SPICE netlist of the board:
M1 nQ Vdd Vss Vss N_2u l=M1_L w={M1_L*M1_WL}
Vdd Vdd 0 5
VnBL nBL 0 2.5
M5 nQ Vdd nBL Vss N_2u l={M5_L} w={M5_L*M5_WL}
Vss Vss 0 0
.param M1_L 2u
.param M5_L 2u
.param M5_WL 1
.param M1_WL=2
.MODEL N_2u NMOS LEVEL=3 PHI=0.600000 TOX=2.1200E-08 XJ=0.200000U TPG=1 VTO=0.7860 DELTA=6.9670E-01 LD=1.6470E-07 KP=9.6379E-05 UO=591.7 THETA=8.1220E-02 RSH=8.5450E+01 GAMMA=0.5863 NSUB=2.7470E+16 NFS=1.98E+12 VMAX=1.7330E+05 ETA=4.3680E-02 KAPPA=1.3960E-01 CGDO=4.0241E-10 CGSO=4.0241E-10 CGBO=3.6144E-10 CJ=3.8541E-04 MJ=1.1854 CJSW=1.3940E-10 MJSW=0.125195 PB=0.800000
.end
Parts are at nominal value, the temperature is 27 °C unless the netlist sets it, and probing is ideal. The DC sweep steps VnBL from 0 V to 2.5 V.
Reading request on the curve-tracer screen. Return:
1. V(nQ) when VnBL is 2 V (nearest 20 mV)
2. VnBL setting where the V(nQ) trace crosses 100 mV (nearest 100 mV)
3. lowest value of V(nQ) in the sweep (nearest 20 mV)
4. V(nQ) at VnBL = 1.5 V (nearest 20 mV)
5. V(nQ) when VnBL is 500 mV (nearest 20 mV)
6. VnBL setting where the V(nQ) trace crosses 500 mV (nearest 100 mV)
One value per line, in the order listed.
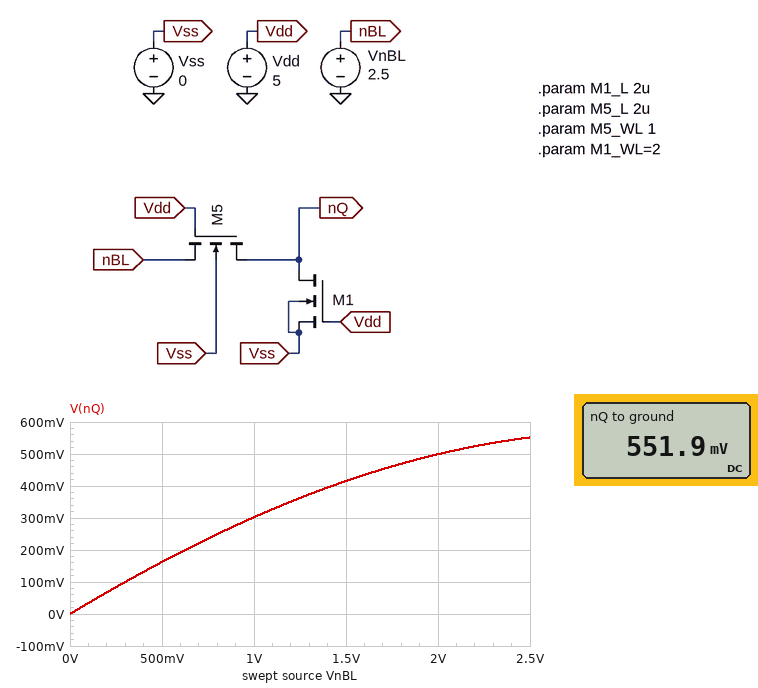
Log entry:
500 mV
300 mV
0 V
420 mV
160 mV
2.0 V
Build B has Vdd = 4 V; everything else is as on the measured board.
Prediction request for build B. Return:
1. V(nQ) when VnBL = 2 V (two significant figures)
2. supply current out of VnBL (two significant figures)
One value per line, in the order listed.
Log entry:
430 mV
210 µA
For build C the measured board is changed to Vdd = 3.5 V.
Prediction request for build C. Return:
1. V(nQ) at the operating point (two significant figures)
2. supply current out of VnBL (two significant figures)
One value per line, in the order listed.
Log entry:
380 mV
160 µA
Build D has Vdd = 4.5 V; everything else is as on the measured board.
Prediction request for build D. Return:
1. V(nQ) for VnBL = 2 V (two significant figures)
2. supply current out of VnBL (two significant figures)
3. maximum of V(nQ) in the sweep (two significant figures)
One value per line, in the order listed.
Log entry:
470 mV
260 µA
500 mV
